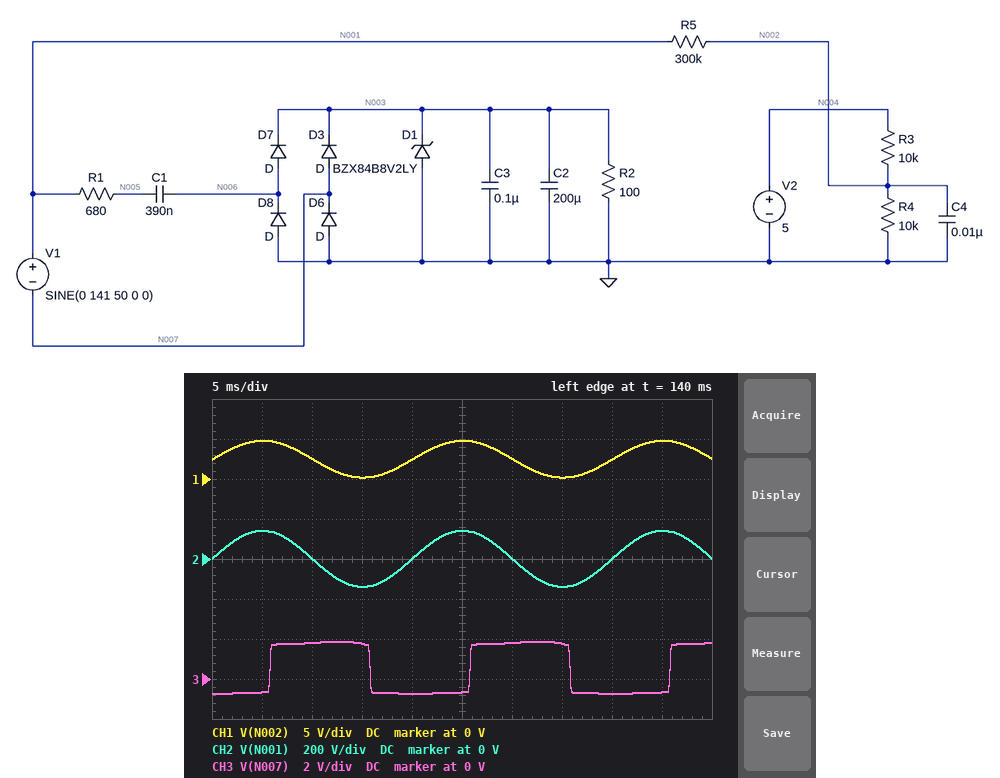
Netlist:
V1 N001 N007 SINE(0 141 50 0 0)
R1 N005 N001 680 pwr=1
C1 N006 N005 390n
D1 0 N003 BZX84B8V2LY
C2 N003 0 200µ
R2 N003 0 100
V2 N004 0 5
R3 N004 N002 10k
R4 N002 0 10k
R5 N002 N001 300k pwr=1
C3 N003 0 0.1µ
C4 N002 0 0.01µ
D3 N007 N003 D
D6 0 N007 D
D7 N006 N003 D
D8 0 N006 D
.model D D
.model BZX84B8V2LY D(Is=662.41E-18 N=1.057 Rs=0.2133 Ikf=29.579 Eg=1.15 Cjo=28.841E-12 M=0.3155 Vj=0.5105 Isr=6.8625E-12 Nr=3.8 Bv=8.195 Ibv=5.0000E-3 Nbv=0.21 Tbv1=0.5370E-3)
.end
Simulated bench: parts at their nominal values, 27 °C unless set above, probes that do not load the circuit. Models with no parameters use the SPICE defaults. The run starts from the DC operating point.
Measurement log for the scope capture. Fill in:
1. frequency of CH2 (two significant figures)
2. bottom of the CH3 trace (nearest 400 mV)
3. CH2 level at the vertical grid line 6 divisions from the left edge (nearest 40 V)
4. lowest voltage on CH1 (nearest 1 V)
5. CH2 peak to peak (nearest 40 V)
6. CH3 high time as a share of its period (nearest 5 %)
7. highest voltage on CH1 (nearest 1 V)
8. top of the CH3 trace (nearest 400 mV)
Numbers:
50 Hz
-800 mV
0 V
0 V
280 V
50 %
5 V
2.0 V
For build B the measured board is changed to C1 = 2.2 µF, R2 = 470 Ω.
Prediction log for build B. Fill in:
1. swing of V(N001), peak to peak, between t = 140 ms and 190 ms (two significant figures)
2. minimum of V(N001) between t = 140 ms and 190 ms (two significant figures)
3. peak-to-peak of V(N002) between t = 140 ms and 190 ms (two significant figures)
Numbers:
270 V
-130 V
4.5 V
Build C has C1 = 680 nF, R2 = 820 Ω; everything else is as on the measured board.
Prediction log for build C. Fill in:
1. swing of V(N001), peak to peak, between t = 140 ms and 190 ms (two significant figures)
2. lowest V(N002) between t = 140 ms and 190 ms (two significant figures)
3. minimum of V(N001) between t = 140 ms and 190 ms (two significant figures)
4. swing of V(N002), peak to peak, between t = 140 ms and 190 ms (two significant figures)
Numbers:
270 V
290 mV
-130 V
4.5 V
